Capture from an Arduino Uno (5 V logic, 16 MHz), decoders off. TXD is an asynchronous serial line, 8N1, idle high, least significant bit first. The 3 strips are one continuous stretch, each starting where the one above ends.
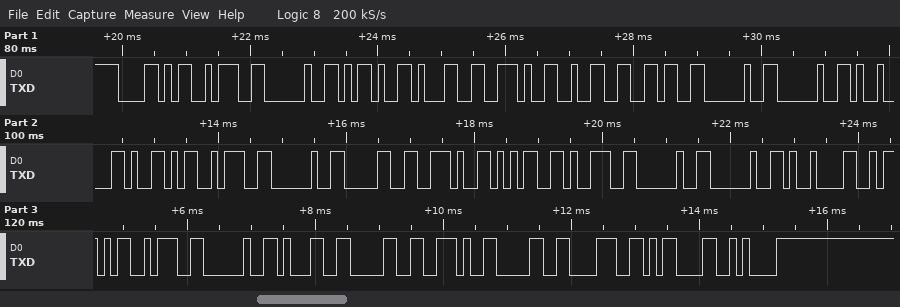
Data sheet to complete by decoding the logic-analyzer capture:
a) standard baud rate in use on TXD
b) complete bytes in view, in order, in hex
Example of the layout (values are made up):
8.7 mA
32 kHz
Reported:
9600 baud
58 3A 20 2D 31 2E 32 36 20 20 09 59 3A 20 30 2E 35 39 20 20 09 5A 3A 20 31 30 2E 30 38 0D 0A
